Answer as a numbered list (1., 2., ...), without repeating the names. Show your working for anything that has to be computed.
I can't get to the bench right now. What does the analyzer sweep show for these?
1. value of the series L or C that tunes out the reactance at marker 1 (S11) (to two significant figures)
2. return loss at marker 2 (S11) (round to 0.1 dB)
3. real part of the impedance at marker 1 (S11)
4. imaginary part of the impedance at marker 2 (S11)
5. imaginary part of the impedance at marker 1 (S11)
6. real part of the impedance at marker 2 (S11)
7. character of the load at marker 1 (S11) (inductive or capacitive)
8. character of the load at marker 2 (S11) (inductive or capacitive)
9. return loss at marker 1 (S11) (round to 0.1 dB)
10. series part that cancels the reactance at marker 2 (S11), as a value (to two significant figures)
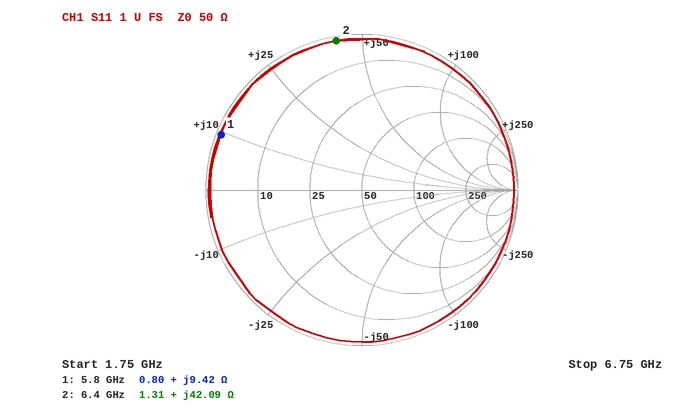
1. C = 1/(2π × 5.8 GHz × 9.42 Ω) ≈ 2.9 pF
2. 0.3 dB
3. 0.80 Ω
4. +42.09 Ω
5. +9.42 Ω
6. 1.31 Ω
7. inductive
8. inductive
9. 0.3 dB
10. C = 1/(2π × 6.4 GHz × 42.09 Ω) ≈ 591 fF, so 590 fF to two significant figures
